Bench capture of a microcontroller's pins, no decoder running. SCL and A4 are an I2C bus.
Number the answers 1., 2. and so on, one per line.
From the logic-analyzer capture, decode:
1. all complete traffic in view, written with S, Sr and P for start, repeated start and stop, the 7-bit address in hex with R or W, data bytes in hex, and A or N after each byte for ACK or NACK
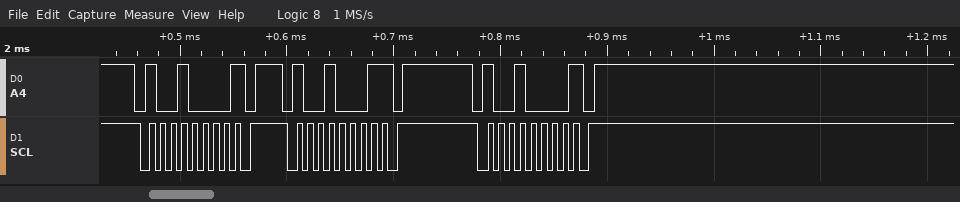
1. S 48W N P S 48R N P S 48W N P
